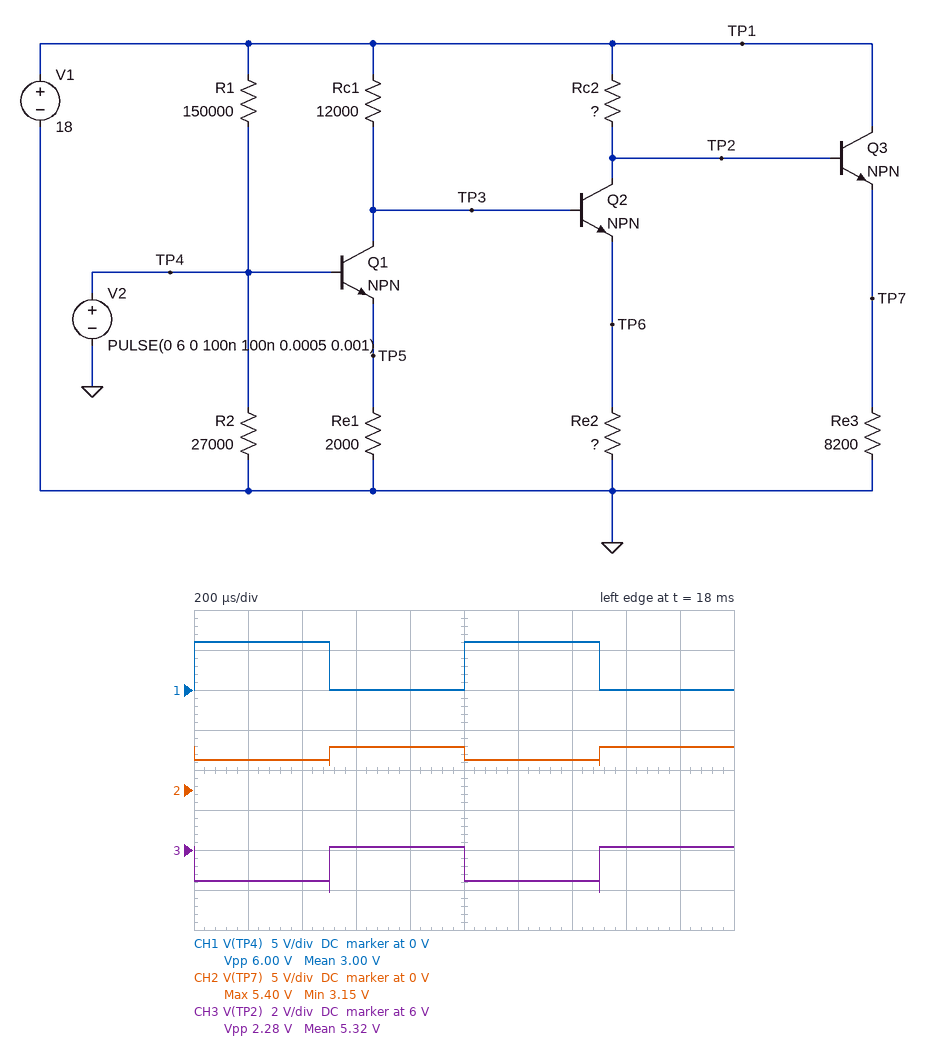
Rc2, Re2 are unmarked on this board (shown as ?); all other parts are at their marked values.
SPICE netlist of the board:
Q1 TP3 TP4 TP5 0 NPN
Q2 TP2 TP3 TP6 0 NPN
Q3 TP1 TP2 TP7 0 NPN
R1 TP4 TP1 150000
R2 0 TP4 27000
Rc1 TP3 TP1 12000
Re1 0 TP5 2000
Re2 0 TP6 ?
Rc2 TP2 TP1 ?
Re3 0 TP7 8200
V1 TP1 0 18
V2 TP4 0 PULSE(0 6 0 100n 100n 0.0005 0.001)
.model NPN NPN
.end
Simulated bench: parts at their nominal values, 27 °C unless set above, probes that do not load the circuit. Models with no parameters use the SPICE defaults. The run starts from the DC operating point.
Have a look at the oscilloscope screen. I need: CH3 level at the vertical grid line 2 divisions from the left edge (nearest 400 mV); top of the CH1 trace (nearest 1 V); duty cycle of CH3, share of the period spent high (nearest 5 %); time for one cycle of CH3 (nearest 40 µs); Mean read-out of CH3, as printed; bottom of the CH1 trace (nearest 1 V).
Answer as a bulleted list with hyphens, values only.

- 4.4 V
- 6 V
- 50 %
- 1.00 ms
- 5.32 V
- 0 V
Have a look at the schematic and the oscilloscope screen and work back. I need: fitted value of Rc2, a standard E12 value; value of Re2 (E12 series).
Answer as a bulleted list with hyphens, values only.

- 18 kΩ
- 3.9 kΩ
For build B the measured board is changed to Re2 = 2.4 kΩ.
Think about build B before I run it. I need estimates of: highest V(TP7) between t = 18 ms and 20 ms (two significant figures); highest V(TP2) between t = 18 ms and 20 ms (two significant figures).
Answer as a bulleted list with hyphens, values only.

- 3.7 V
- 4.4 V
